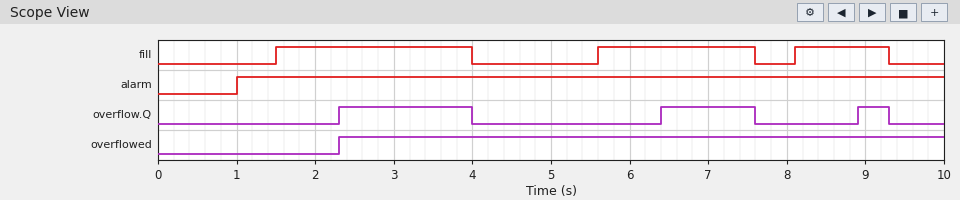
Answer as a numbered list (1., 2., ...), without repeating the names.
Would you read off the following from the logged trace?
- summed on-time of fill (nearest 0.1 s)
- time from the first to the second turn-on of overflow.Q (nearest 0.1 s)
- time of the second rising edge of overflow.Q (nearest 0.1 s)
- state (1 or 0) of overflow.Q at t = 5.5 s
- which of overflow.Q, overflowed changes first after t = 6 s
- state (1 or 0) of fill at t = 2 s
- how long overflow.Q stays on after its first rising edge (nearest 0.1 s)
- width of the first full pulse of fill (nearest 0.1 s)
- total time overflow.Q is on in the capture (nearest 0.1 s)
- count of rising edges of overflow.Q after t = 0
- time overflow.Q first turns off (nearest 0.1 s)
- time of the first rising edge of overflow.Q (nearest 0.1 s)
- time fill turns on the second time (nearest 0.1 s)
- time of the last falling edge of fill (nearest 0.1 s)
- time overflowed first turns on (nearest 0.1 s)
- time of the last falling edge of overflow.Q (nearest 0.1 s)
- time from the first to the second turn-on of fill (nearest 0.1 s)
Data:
1. 5.7 s
2. 4.1 s
3. 6.4 s
4. 0
5. overflow.Q
6. 1
7. 1.7 s
8. 2.5 s
9. 3.3 s
10. 3
11. 4.0 s
12. 2.3 s
13. 5.6 s
14. 9.3 s
15. 2.3 s
16. 9.3 s
17. 4.1 s
